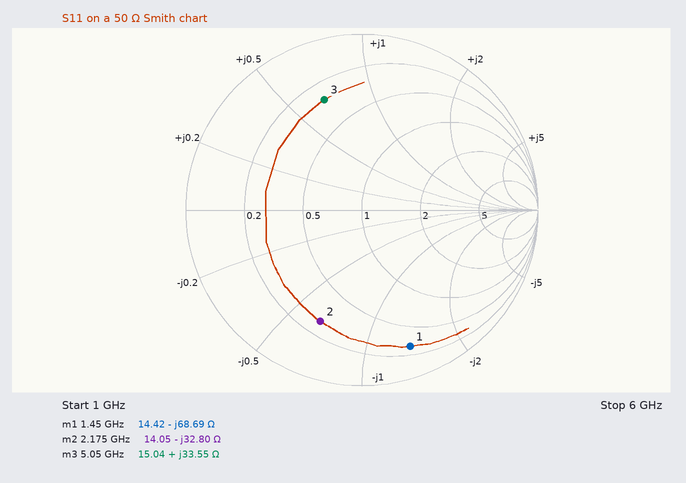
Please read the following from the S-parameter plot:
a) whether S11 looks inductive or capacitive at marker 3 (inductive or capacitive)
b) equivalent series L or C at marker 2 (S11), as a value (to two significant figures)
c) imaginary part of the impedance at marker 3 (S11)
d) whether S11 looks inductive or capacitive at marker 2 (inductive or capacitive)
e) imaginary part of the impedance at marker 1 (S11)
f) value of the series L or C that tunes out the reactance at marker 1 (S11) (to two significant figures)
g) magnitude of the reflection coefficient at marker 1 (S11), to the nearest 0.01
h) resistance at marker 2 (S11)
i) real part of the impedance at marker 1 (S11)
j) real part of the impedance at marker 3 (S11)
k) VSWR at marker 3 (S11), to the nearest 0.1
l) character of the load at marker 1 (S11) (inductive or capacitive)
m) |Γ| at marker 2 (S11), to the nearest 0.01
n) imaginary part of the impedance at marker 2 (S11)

inductive
2.2 pF
+33.55 Ω
capacitive
-68.69 Ω
7.5 nH
0.82
14.05 Ω
14.42 Ω
15.04 Ω
4.9
capacitive
0.68
-32.80 Ω
